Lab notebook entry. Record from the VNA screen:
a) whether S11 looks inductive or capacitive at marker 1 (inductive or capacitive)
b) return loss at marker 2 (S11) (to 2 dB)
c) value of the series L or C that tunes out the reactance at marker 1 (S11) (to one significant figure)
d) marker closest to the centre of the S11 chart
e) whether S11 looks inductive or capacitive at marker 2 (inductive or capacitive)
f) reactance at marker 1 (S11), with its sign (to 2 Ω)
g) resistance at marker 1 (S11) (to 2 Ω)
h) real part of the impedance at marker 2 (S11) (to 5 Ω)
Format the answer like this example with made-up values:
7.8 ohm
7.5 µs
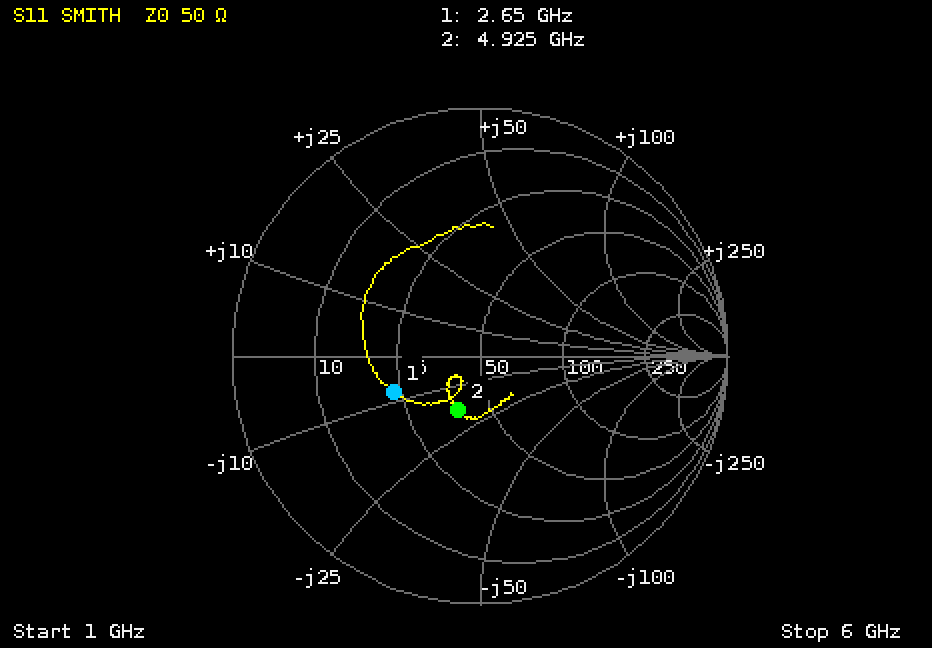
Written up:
capacitive
12 dB
500 pH
marker 2
capacitive
-8 Ω
24 Ω
40 Ω
